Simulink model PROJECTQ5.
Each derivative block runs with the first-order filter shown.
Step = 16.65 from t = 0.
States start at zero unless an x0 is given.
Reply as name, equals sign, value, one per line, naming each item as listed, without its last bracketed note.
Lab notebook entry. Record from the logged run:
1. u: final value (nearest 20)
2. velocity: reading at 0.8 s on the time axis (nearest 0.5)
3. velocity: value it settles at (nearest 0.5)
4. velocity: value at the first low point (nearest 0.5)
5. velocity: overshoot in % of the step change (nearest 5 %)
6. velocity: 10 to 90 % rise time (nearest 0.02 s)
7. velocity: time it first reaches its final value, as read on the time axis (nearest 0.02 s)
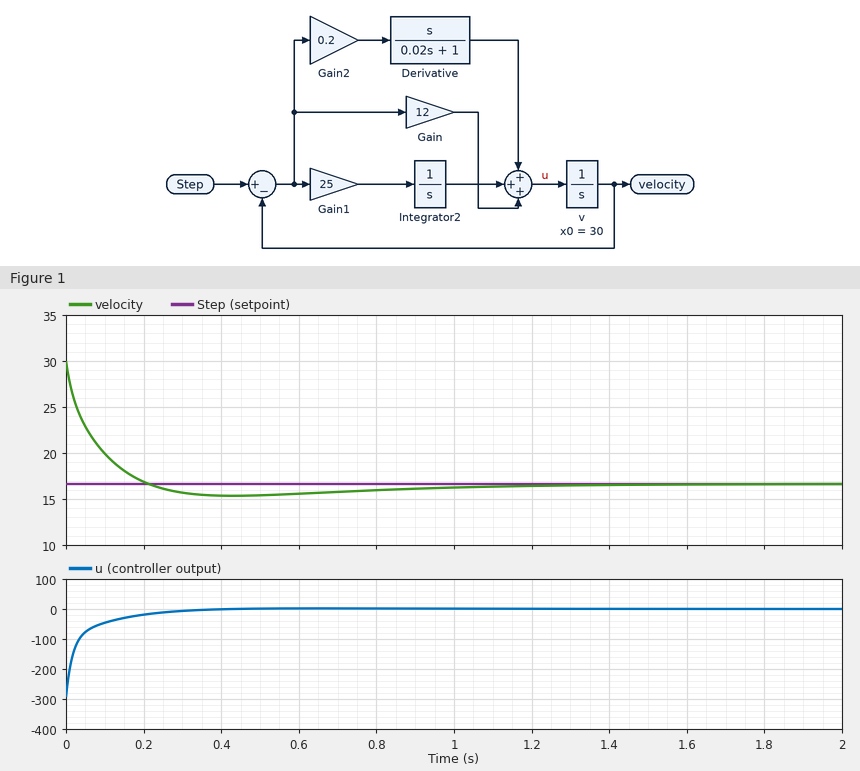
u: final value = 0
velocity: reading at 0.8 s on the time axis = 16.0
velocity: value it settles at = 16.5
velocity: value at the first low point = 15.5
velocity: overshoot in % of the step change = 10 %
velocity: 10 to 90 % rise time = 0.14 s
velocity: time it first reaches its final value, as read on the time axis = 0.22 s
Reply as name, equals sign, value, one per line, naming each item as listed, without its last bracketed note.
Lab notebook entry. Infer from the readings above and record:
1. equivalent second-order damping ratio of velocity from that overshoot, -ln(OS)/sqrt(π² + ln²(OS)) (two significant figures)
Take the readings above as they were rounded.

equivalent second-order damping ratio of velocity from that overshoot, -ln(OS)/sqrt(π² + ln²(OS)) = 0.59
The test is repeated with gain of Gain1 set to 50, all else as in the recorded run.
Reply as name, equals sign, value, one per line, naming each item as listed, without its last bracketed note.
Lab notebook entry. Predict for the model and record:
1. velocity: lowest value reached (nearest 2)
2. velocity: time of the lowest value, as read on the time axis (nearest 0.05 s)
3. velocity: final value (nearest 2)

velocity: lowest value reached = 14
velocity: time of the lowest value, as read on the time axis = 0.35 s
velocity: final value = 16
